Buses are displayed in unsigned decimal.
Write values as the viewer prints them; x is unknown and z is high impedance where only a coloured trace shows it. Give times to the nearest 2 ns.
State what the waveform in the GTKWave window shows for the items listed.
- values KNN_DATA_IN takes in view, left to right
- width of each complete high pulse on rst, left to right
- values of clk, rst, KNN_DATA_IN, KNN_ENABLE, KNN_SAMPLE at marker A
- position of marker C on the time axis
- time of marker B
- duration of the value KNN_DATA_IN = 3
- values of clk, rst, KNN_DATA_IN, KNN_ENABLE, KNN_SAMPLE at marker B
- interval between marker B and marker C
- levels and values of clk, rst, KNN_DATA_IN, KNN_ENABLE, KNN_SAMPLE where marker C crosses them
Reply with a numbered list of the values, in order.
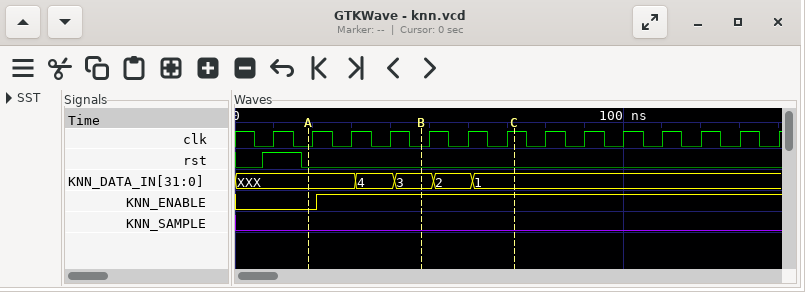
1. XXX, 4, 3, 2, 1
2. 10 ns
3. clk=0, rst=0, KNN_DATA_IN=XXX, KNN_ENABLE=0, KNN_SAMPLE=0
4. 72 ns
5. 48 ns
6. 10 ns
7. clk=0, rst=0, KNN_DATA_IN=3, KNN_ENABLE=1, KNN_SAMPLE=0
8. 24 ns
9. clk=1, rst=0, KNN_DATA_IN=1, KNN_ENABLE=1, KNN_SAMPLE=0
